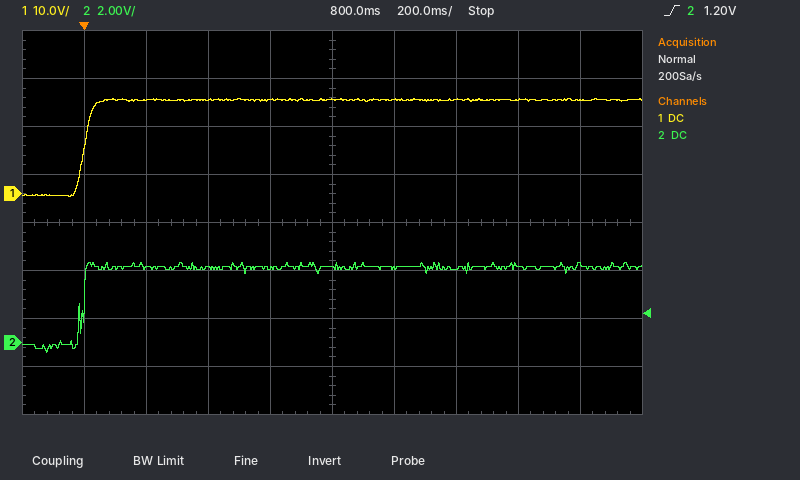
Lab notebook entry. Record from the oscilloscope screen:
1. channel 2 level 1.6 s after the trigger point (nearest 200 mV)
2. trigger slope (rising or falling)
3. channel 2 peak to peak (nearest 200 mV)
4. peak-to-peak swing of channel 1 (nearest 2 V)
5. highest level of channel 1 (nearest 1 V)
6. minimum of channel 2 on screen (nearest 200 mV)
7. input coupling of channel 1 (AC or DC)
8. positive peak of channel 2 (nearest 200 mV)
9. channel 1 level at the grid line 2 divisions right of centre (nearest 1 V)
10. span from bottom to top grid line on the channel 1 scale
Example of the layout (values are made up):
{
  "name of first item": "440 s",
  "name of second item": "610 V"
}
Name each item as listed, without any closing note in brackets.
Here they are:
{
  "channel 2 level 1.6 s after the trigger point": "3.2 V",
  "trigger slope": "rising",
  "channel 2 peak to peak": "3.8 V",
  "peak-to-peak swing of channel 1": "20 V",
  "highest level of channel 1": "20 V",
  "minimum of channel 2 on screen": "-400 mV",
  "input coupling of channel 1": "DC",
  "positive peak of channel 2": "3.4 V",
  "channel 1 level at the grid line 2 divisions right of centre": "20 V",
  "span from bottom to top grid line on the channel 1 scale": "80 V"
}
